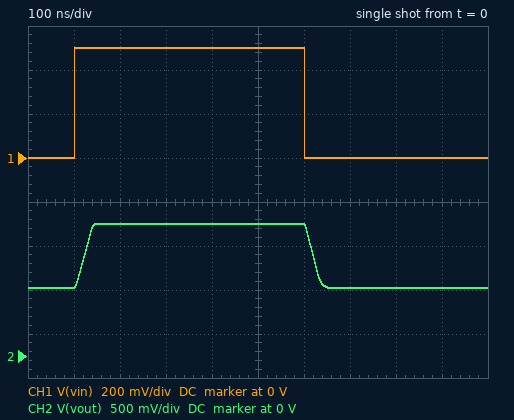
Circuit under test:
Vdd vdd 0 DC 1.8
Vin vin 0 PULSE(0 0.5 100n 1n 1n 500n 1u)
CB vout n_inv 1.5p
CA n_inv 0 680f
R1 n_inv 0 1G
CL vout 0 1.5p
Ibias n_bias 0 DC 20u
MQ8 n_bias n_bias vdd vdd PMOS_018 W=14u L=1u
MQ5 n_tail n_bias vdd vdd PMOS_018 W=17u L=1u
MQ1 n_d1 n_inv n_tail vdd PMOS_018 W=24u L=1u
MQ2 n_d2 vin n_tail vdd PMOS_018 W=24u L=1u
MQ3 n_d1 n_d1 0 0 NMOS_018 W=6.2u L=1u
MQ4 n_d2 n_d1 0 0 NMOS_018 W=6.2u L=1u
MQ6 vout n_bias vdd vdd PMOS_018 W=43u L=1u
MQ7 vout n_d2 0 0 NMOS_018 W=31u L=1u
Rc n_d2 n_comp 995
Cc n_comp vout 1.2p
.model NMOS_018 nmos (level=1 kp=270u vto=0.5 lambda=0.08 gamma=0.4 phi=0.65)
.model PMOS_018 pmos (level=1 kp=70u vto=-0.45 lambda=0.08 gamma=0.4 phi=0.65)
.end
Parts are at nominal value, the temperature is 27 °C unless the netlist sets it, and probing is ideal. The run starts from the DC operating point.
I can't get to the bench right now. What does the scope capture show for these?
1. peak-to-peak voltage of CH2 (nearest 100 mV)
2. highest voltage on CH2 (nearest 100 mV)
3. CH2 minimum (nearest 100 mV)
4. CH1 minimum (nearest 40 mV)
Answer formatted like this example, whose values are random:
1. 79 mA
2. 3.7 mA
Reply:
1. 700 mV
2. 1.5 V
3. 800 mV
4. 0 V
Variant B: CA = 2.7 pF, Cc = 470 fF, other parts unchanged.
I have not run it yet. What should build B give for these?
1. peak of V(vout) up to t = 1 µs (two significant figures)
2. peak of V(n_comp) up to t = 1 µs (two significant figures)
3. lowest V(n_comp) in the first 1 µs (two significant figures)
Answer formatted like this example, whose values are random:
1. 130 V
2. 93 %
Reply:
1. 1.8 V
2. 690 mV
3. 3.4 mV
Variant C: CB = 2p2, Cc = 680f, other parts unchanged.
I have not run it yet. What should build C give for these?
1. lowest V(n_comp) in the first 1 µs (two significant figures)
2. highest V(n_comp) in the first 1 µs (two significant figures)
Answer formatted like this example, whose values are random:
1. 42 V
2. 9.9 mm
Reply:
1. 140 mV
2. 660 mV
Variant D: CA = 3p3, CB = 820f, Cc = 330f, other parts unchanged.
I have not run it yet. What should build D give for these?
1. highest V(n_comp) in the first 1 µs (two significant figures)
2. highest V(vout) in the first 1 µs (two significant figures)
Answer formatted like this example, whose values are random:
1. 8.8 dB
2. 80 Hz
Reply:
1. 700 mV
2. 1.8 V
